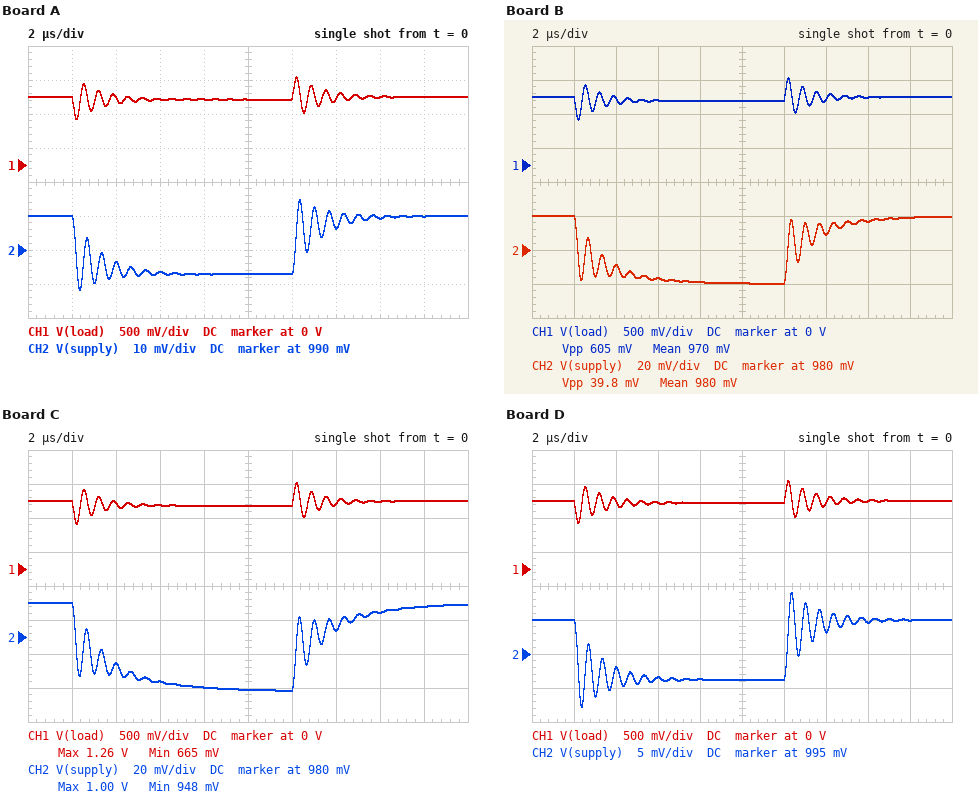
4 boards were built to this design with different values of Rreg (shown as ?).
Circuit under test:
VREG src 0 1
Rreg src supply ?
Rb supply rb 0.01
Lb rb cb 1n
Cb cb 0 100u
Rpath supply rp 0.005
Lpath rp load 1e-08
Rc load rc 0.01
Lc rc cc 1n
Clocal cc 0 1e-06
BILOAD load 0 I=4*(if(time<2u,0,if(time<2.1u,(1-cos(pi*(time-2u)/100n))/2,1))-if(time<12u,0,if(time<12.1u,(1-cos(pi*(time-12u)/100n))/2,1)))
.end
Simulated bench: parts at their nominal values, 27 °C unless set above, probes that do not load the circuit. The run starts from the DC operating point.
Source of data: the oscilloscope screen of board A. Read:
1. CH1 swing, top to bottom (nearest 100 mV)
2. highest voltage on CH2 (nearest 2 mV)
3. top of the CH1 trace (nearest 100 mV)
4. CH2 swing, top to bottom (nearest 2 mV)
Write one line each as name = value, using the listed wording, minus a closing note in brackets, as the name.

CH1 swing, top to bottom = 600 mV
highest voltage on CH2 = 1.004 V
top of the CH1 trace = 1.3 V
CH2 swing, top to bottom = 26 mV
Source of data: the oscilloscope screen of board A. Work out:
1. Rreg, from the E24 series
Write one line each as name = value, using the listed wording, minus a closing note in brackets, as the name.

Rreg, from the E24 series = 4.3 mΩ
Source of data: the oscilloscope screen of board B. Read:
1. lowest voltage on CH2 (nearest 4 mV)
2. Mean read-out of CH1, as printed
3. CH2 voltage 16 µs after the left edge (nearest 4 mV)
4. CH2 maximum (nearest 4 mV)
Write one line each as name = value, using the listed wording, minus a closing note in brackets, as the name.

lowest voltage on CH2 = 960 mV
Mean read-out of CH1, as printed = 970 mV
CH2 voltage 16 µs after the left edge = 996 mV
CH2 maximum = 1.000 V
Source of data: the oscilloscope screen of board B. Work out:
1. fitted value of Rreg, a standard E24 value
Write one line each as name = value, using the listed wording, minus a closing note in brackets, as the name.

fitted value of Rreg, a standard E24 value = 0.01 Ω
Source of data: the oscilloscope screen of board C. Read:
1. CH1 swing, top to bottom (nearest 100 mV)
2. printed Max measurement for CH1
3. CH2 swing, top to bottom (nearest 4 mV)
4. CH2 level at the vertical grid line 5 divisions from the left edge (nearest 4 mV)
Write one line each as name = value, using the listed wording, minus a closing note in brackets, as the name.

CH1 swing, top to bottom = 600 mV
printed Max measurement for CH1 = 1.26 V
CH2 swing, top to bottom = 52 mV
CH2 level at the vertical grid line 5 divisions from the left edge = 948 mV
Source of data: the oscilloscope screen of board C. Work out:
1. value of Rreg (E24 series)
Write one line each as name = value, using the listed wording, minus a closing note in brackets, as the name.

value of Rreg = 0.013 Ω
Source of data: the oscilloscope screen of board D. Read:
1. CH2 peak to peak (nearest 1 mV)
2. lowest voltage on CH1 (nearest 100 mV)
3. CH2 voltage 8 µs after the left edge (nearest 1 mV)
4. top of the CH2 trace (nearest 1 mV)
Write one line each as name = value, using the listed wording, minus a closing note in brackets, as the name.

CH2 peak to peak = 17 mV
lowest voltage on CH1 = 700 mV
CH2 voltage 8 µs after the left edge = 991 mV
top of the CH2 trace = 1.004 V
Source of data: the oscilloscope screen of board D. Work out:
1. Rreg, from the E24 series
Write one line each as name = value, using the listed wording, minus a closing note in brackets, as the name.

Rreg, from the E24 series = 2.2 mΩ
